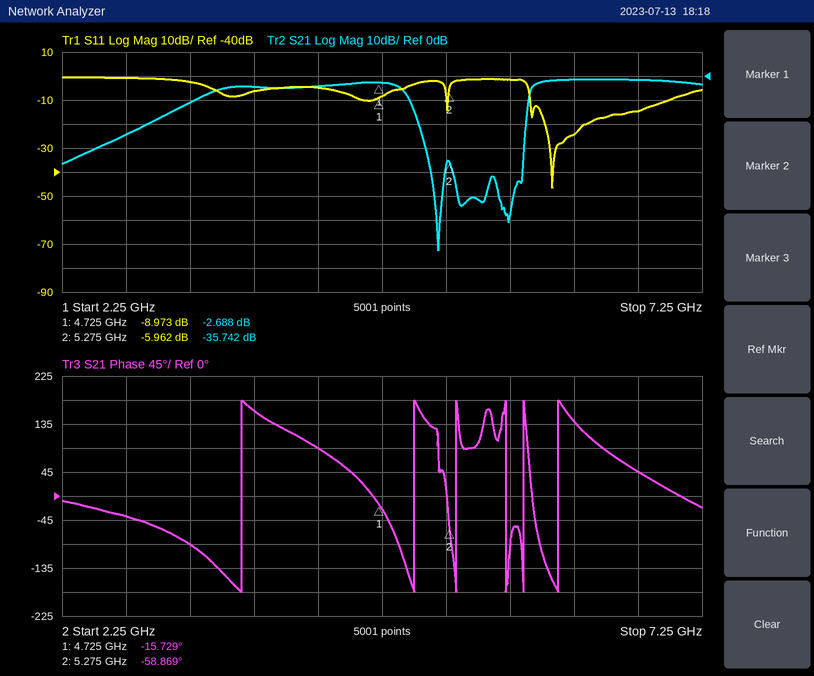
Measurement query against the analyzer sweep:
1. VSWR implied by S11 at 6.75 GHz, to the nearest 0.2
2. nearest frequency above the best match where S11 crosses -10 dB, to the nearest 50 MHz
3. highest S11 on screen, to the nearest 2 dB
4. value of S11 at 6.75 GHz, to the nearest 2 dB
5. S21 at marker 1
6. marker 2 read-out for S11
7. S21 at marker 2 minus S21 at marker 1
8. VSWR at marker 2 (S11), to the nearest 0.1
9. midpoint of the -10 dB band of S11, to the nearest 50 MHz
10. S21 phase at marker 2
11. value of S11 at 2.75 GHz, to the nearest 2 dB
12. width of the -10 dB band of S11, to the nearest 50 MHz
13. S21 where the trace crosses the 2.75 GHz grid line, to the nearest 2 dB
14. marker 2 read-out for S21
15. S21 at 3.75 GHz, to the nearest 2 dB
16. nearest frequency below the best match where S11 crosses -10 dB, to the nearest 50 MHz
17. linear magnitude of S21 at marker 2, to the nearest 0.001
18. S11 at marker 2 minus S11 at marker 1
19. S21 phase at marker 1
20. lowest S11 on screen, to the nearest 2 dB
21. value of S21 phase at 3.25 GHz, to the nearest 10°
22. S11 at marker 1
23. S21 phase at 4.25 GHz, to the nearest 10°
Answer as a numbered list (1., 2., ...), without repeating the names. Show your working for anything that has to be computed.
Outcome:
1. |Γ| = 10^(-14/20) = 0.1995; VSWR = (1 + 0.1995)/(1 − 0.1995) ≈ 1.50, so 1.4 to the nearest 0.2
2. 7.00 GHz
3. 0 dB
4. -14 dB
5. -2.688 dB
6. -5.962 dB
7. -35.742 − (-2.688) = -33.054 dB
8. (1 + 0.5034)/(1 − 0.5034) ≈ 3.0
9. 6.45 GHz
10. -58.869°
11. 0 dB
12. 7.00 GHz − 5.90 GHz = 1.10 GHz
13. -24 dB
14. -35.742 dB
15. -4 dB
16. 5.90 GHz
17. 10^(-35.742/20) ≈ 0.016
18. -5.962 − (-8.973) = 3.011 dB
19. -15.729°
20. -46 dB
21. -90°
22. -8.973 dB
23. 90°
